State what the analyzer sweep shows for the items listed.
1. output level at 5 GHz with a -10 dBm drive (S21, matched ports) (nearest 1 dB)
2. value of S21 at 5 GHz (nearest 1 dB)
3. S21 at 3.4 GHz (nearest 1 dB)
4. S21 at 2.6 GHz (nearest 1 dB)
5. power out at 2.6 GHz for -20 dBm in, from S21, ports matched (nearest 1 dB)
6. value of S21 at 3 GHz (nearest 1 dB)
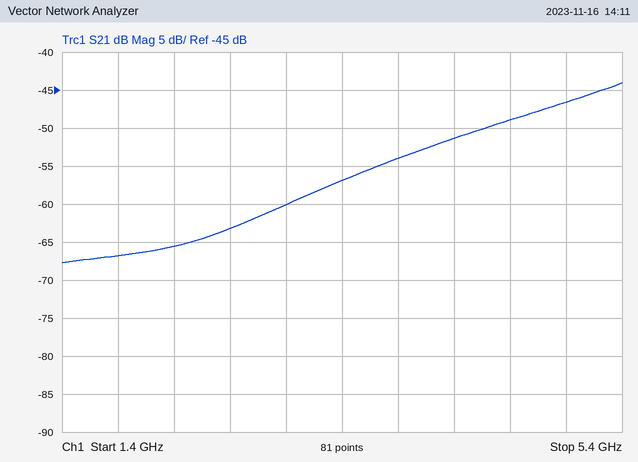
-57 dBm
-47 dB
-57 dB
-63 dB
-83 dBm
-60 dB
